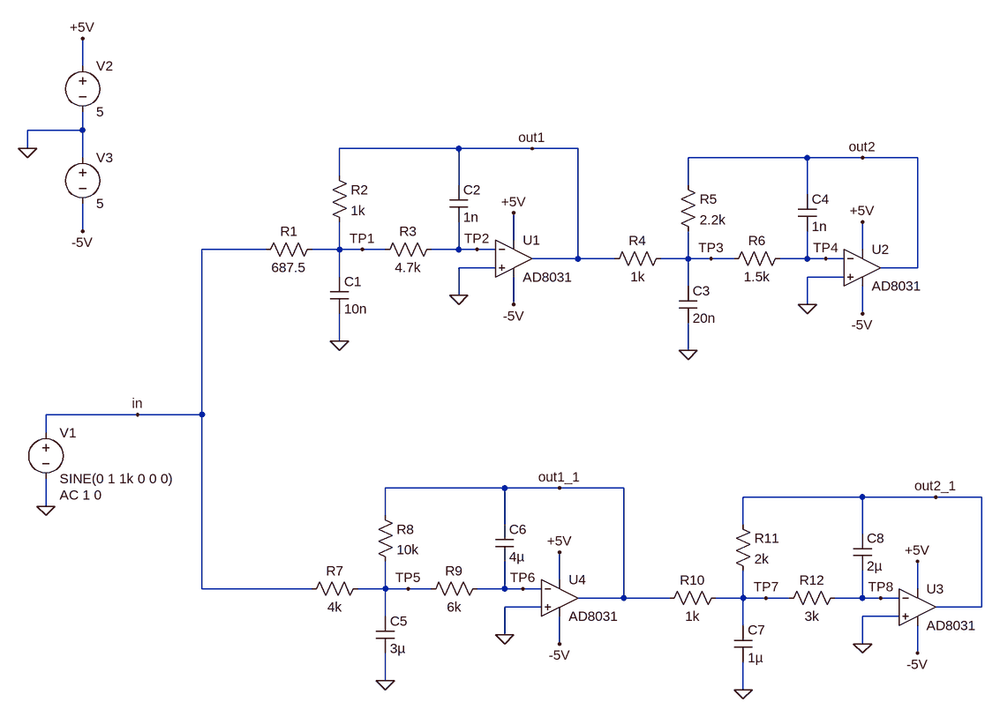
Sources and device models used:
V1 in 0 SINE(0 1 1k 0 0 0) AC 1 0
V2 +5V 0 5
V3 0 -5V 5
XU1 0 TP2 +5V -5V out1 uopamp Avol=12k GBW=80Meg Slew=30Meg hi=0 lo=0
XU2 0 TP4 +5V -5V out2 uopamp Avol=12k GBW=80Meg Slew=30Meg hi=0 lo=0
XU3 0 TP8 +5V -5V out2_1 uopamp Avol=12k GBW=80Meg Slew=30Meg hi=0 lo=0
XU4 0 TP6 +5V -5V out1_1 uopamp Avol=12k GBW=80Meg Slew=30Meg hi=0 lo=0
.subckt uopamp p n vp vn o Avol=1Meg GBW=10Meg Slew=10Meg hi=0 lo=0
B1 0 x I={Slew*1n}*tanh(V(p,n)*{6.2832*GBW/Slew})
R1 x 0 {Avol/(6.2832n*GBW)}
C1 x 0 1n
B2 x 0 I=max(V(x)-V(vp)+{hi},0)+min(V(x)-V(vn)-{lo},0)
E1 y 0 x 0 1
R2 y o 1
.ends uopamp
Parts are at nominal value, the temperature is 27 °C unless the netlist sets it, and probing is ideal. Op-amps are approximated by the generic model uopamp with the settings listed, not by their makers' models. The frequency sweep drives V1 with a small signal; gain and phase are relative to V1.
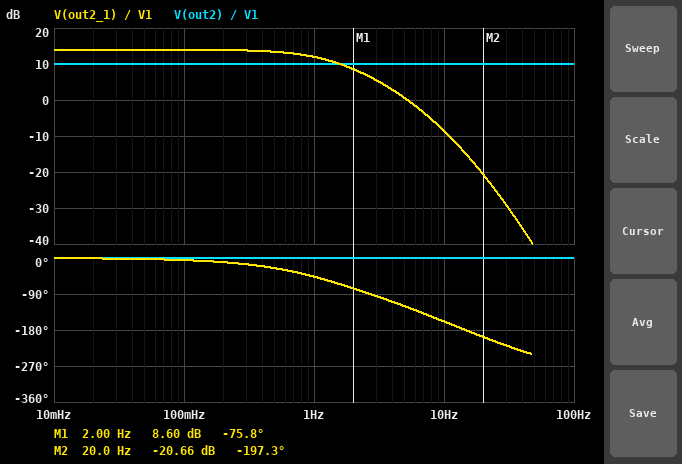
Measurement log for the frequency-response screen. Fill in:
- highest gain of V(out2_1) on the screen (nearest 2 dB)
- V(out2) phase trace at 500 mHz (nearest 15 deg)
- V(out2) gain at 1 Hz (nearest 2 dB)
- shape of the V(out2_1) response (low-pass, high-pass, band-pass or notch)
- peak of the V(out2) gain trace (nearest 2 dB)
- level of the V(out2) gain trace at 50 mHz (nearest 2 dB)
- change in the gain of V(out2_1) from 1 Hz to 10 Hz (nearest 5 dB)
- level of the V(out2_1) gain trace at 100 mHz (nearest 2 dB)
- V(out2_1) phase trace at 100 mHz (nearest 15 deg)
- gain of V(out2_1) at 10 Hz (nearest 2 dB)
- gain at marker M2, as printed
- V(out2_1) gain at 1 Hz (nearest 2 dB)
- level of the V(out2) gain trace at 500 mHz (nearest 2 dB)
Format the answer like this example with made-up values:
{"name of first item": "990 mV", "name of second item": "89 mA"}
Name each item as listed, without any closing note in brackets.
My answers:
{"highest gain of V(out2_1) on the screen": "14 dB", "V(out2) phase trace at 500 mHz": "0 deg", "V(out2) gain at 1 Hz": "10 dB", "shape of the V(out2_1) response": "low-pass", "peak of the V(out2) gain trace": "10 dB", "level of the V(out2) gain trace at 50 mHz": "10 dB", "change in the gain of V(out2_1) from 1 Hz to 10 Hz": "-20 dB", "level of the V(out2_1) gain trace at 100 mHz": "14 dB", "V(out2_1) phase trace at 100 mHz": "0 deg", "gain of V(out2_1) at 10 Hz": "-8 dB", "gain at marker M2, as printed": "-20.66 dB", "V(out2_1) gain at 1 Hz": "12 dB", "level of the V(out2) gain trace at 500 mHz": "10 dB"}
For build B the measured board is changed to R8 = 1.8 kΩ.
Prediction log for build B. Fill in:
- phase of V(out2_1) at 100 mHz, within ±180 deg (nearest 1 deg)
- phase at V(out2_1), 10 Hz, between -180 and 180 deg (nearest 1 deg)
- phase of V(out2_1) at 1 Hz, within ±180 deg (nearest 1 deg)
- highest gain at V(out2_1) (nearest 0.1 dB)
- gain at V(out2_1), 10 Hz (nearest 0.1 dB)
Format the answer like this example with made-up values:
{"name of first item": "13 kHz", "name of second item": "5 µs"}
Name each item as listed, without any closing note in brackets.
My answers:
{"phase of V(out2_1) at 100 mHz, within ±180 deg": "-2 deg", "phase at V(out2_1), 10 Hz, between -180 and 180 deg": "-135 deg", "phase of V(out2_1) at 1 Hz, within ±180 deg": "-23 deg", "highest gain at V(out2_1)": "-0.9 dB", "gain at V(out2_1), 10 Hz": "-14.0 dB"}
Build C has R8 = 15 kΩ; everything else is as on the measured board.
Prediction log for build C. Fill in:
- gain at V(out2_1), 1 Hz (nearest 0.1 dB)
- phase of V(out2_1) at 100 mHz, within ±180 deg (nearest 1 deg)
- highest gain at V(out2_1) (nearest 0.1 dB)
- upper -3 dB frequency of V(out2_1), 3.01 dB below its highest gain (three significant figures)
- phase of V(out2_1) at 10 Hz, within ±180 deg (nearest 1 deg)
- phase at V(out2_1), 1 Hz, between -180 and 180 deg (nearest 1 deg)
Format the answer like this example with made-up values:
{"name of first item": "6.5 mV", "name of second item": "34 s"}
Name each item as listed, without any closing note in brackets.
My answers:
{"gain at V(out2_1), 1 Hz": "14.2 dB", "phase of V(out2_1) at 100 mHz, within ±180 deg": "-7 deg", "highest gain at V(out2_1)": "17.5 dB", "upper -3 dB frequency of V(out2_1), 3.01 dB below its highest gain": "934 mHz", "phase of V(out2_1) at 10 Hz, within ±180 deg": "-162 deg", "phase at V(out2_1), 1 Hz, between -180 and 180 deg": "-57 deg"}
